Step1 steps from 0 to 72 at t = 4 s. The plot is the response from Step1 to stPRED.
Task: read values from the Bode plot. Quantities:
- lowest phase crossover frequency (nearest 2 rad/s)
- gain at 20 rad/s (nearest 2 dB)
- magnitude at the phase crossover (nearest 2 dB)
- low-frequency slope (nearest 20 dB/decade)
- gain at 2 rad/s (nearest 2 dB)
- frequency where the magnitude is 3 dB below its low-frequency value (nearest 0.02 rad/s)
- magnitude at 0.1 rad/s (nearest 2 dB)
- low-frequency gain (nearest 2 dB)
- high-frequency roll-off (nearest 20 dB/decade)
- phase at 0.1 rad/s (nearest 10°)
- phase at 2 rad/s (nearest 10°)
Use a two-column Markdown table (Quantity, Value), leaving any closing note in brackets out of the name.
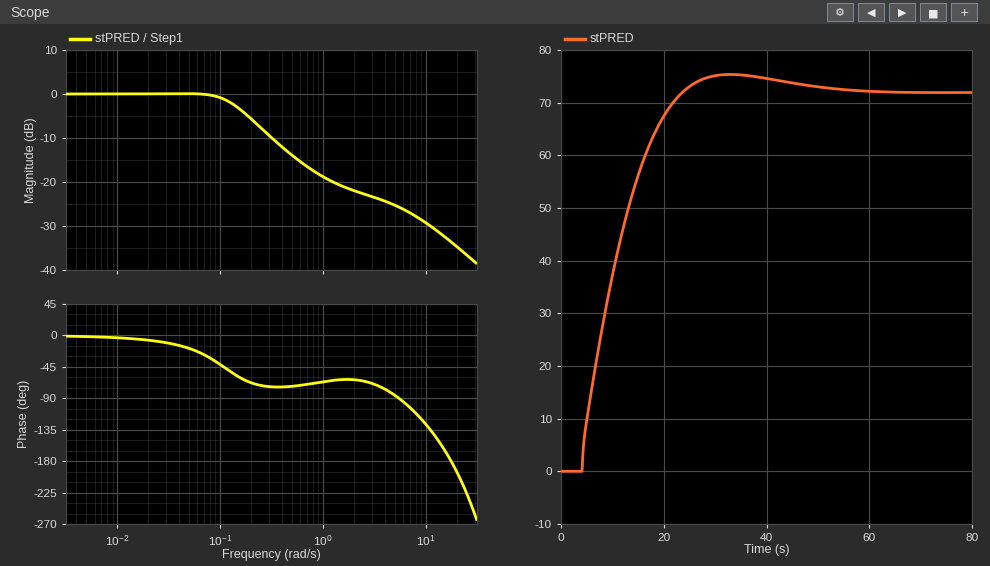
| Quantity | Value |
|---|---|
| lowest phase crossover frequency | 18 rad/s |
| gain at 20 rad/s | -34 dB |
| magnitude at the phase crossover | -34 dB |
| low-frequency slope | 0 dB/decade |
| gain at 2 rad/s | -22 dB |
| frequency where the magnitude is 3 dB below its low-frequency value | 0.14 rad/s |
| magnitude at 0.1 rad/s | 0 dB |
| low-frequency gain | 0 dB |
| high-frequency roll-off | -20 dB/decade |
| phase at 0.1 rad/s | -40° |
| phase at 2 rad/s | -60° |
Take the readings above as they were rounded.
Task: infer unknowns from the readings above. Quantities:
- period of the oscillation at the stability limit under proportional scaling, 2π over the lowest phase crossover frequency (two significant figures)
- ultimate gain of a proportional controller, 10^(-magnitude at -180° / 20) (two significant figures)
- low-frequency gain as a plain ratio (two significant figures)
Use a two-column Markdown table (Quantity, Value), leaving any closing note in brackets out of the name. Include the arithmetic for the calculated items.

| Quantity | Value |
|---|---|
| period of the oscillation at the stability limit under proportional scaling, 2π over the lowest phase crossover frequency | 2π / 18 = 0.35 s |
| ultimate gain of a proportional controller, 10^(-magnitude at -180° / 20) | 10^(34 / 20) = 50 |
| low-frequency gain as a plain ratio | 10^(0 / 20) = 1.0 |
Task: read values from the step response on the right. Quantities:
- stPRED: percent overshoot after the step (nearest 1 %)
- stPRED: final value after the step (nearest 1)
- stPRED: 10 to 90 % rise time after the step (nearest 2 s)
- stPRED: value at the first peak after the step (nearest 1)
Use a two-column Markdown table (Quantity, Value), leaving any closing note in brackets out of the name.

| Quantity | Value |
|---|---|
| stPRED: percent overshoot after the step | 5 % |
| stPRED: final value after the step | 72 |
| stPRED: 10 to 90 % rise time after the step | 14 s |
| stPRED: value at the first peak after the step | 75 |
